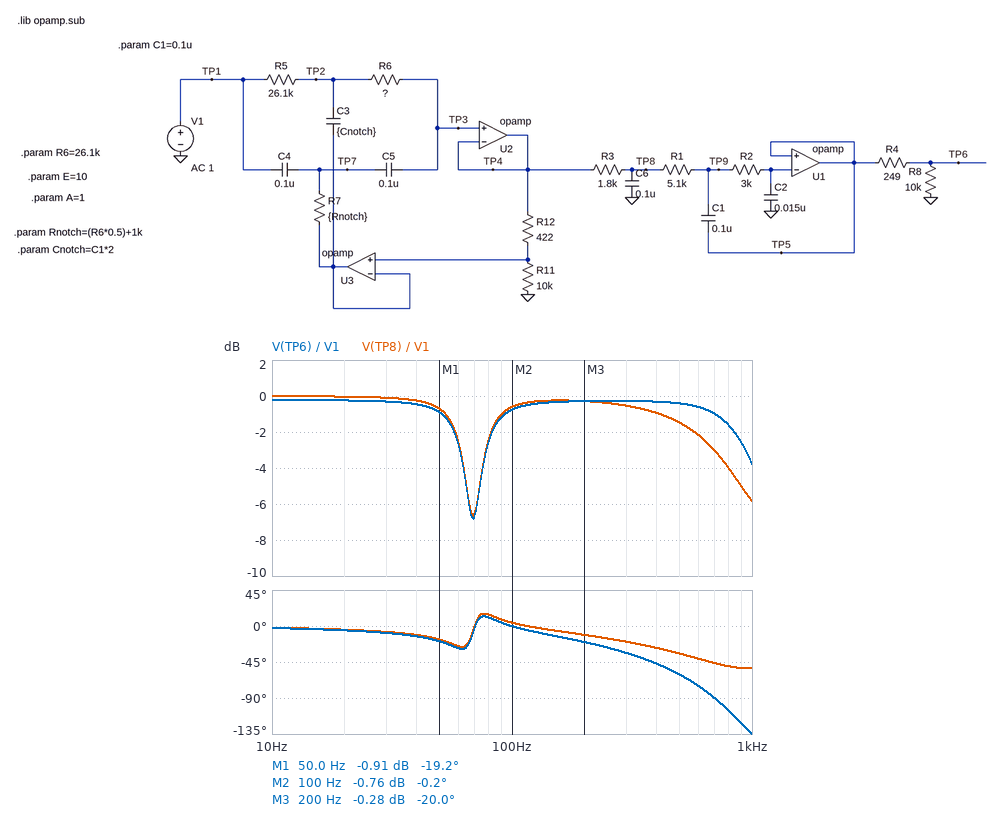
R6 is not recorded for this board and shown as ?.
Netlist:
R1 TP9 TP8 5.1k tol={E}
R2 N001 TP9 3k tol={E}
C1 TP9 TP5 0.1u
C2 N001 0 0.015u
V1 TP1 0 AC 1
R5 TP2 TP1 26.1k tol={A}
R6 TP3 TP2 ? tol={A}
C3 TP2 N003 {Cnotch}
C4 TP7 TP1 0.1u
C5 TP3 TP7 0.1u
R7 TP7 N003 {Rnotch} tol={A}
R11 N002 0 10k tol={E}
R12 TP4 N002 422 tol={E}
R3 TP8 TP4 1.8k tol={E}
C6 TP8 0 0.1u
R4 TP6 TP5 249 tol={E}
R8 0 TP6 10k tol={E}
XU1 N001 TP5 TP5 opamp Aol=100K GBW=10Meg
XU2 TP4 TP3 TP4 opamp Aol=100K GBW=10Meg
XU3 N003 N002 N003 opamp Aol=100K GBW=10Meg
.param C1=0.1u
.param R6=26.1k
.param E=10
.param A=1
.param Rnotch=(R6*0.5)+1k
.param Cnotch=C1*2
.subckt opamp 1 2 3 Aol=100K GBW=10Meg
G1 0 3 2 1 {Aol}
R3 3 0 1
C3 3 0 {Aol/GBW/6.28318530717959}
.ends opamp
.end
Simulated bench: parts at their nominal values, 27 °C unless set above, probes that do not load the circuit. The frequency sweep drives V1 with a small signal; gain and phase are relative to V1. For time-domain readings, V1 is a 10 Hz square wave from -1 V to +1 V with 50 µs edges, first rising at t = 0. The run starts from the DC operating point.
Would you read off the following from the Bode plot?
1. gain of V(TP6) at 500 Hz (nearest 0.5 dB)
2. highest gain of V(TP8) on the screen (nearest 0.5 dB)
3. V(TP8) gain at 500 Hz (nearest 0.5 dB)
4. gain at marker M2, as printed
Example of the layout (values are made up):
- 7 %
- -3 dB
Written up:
- -0.5 dB
- 0 dB
- -1.5 dB
- -0.76 dB
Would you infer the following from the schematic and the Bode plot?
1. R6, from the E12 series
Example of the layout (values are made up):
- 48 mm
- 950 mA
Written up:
- 18 kΩ
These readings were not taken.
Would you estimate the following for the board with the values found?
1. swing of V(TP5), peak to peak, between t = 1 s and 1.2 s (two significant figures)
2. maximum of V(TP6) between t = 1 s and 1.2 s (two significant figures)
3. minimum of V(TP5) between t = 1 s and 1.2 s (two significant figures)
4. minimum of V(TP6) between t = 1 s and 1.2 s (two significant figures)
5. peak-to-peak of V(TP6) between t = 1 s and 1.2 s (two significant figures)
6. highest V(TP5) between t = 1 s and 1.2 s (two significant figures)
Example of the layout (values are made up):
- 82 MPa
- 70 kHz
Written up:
- 2.3 V
- 1.1 V
- -1.2 V
- -1.1 V
- 2.3 V
- 1.2 V
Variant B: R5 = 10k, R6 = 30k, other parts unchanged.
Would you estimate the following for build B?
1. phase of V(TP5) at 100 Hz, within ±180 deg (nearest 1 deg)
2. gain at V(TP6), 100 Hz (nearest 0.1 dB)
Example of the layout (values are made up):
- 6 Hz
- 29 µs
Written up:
- -4 deg
- -1.2 dB
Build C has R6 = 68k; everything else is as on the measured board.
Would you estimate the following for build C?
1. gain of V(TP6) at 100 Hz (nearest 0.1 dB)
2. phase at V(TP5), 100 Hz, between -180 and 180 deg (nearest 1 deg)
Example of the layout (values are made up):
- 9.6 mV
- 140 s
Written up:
- -0.2 dB
- -7 deg
